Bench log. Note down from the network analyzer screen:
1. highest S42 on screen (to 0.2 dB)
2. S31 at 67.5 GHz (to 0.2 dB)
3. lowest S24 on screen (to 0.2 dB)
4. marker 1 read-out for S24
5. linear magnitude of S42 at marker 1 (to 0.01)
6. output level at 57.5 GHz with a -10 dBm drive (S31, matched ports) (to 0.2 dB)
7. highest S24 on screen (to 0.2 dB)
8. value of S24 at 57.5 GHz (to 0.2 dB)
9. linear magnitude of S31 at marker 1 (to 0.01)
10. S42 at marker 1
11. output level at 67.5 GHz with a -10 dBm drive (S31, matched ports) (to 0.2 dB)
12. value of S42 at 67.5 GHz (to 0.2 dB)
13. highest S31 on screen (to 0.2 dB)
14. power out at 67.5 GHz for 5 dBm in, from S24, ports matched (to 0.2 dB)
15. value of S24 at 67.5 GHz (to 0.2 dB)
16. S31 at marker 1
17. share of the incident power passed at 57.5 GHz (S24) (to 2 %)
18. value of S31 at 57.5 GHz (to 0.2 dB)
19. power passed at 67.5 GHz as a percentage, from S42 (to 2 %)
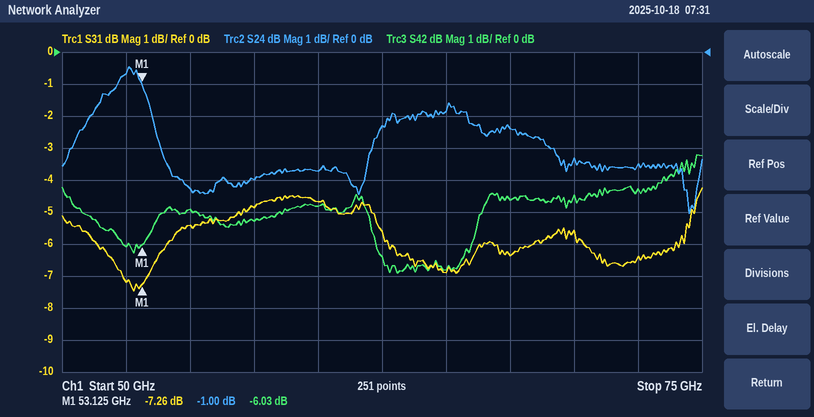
-3.2 dB
-6.4 dB
-5.0 dB
-1.00 dB
0.50
-14.8 dBm
-0.4 dB
-4.0 dB
0.43
-6.03 dB
-16.4 dBm
-4.6 dB
-4.2 dB
2.6 dBm
-2.4 dB
-7.26 dB
40 %
-4.8 dB
34 %
